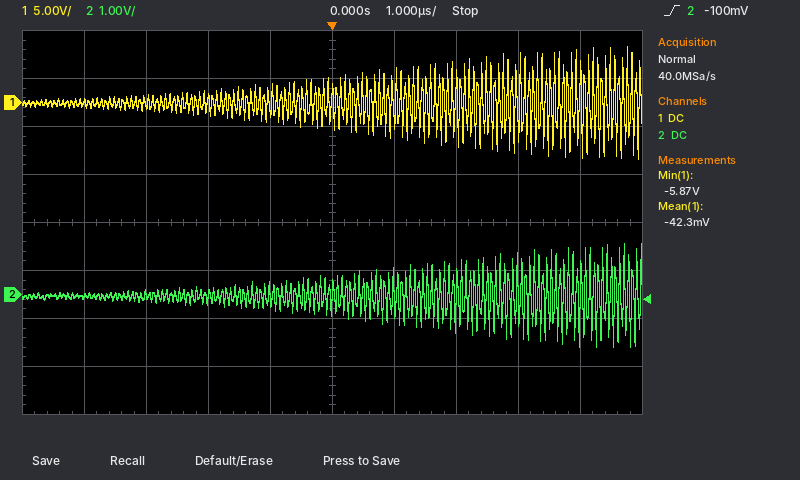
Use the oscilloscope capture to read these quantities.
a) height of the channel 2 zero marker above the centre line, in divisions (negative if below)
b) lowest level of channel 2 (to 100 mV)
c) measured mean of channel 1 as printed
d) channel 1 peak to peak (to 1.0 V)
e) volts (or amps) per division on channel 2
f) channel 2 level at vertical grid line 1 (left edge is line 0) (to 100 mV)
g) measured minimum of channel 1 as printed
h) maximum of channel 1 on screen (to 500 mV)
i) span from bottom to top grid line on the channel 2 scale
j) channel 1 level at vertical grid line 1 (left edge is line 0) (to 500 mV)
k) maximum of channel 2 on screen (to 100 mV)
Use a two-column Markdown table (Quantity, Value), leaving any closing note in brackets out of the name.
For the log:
| Quantity | Value |
|---|---|
| height of the channel 2 zero marker above the centre line, in divisions | -1.5 div |
| lowest level of channel 2 | -1.1 V |
| measured mean of channel 1 as printed | -42.3 mV |
| channel 1 peak to peak | 12.0 V |
| volts (or amps) per division on channel 2 | 1 V |
| channel 2 level at vertical grid line 1 (left edge is line 0) | 0.0 V |
| measured minimum of channel 1 as printed | -5.87 V |
| maximum of channel 1 on screen | 6.0 V |
| span from bottom to top grid line on the channel 2 scale | 8 V |
| channel 1 level at vertical grid line 1 (left edge is line 0) | 0.0 V |
| maximum of channel 2 on screen | 1.1 V |
